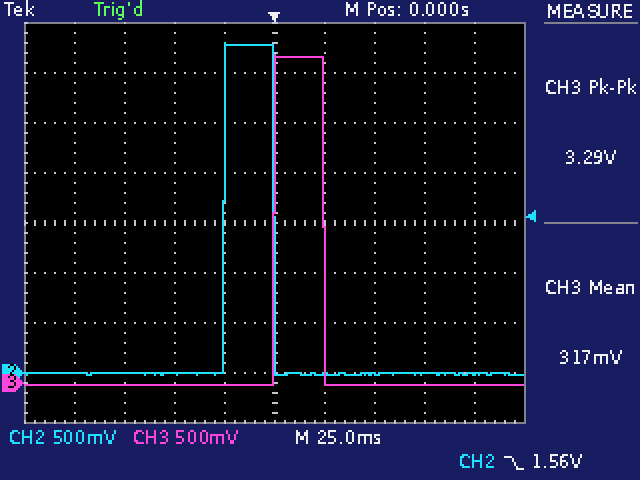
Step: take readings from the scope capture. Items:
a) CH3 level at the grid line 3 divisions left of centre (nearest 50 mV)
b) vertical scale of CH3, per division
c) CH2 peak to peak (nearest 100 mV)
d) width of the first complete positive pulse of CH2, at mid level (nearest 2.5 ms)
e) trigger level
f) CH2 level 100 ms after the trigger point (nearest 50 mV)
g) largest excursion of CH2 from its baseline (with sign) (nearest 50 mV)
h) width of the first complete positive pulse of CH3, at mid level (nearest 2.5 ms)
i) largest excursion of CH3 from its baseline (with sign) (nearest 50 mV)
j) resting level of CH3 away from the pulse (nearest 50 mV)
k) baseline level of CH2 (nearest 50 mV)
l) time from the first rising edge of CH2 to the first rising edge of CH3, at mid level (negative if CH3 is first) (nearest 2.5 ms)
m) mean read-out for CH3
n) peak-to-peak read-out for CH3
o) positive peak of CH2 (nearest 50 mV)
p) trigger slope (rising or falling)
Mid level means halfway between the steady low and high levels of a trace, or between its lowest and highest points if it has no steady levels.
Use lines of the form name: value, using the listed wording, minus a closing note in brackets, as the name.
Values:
CH3 level at the grid line 3 divisions left of centre: 0 mV
vertical scale of CH3, per division: 500 mV
CH2 peak to peak: 3.30 V
width of the first complete positive pulse of CH2, at mid level: 25.0 ms
trigger level: 1.56 V
CH2 level 100 ms after the trigger point: 0 mV
largest excursion of CH2 from its baseline (with sign): +3.30 V
width of the first complete positive pulse of CH3, at mid level: 25.0 ms
largest excursion of CH3 from its baseline (with sign): +3.30 V
resting level of CH3 away from the pulse: 0 mV
baseline level of CH2: 0 mV
time from the first rising edge of CH2 to the first rising edge of CH3, at mid level (negative if CH3 is first): +25.0 ms
mean read-out for CH3: 317 mV
peak-to-peak read-out for CH3: 3.29 V
positive peak of CH2: 3.30 V
trigger slope: falling
